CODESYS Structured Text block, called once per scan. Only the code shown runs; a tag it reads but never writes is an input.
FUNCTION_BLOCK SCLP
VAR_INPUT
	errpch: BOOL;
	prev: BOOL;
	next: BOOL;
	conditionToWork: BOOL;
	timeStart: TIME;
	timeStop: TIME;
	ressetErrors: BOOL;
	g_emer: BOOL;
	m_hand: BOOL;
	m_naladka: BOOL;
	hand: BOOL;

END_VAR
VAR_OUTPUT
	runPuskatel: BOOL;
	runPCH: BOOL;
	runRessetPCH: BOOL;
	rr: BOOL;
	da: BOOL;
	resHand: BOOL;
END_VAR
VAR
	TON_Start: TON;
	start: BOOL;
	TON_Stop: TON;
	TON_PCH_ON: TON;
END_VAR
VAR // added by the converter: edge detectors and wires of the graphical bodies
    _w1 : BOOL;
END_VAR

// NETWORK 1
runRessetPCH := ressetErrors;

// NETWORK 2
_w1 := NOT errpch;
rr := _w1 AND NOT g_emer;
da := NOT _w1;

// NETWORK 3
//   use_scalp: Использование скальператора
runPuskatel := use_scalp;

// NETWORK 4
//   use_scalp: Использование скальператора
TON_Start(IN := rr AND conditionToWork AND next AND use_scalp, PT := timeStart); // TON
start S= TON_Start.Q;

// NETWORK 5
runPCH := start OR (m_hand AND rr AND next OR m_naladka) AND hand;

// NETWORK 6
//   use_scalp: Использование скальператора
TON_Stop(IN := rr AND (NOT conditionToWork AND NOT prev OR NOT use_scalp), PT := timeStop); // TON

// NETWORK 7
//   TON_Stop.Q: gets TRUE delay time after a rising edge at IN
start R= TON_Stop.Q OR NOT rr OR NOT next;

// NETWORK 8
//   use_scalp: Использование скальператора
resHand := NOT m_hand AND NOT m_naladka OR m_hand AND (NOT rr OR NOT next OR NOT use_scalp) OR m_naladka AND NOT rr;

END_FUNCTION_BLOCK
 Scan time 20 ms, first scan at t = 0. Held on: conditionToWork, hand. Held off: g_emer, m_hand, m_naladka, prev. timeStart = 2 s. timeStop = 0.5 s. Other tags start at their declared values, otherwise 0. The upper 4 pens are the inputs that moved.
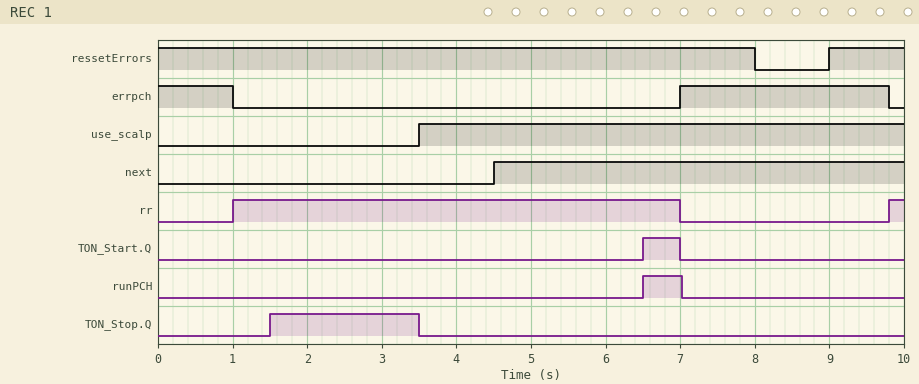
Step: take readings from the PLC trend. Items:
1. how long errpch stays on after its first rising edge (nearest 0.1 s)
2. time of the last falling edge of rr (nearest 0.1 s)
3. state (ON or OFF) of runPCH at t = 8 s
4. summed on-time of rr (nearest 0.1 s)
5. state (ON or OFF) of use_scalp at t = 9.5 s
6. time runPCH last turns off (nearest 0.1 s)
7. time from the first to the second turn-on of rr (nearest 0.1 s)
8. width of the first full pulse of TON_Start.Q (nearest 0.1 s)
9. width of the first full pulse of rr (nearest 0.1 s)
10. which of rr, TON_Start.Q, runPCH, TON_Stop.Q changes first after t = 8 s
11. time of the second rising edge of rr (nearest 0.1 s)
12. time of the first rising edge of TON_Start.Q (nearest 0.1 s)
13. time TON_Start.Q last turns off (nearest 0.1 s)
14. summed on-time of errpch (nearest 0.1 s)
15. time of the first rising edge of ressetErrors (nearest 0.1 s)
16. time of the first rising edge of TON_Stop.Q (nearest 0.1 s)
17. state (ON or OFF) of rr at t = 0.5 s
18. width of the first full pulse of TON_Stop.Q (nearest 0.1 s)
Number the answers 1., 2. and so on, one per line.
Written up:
1. 2.8 s
2. 7.0 s
3. OFF
4. 6.2 s
5. ON
6. 7.0 s
7. 8.8 s
8. 0.5 s
9. 6.0 s
10. rr
11. 9.8 s
12. 6.5 s
13. 7.0 s
14. 3.8 s
15. 9.0 s
16. 1.5 s
17. OFF
18. 2.0 s
